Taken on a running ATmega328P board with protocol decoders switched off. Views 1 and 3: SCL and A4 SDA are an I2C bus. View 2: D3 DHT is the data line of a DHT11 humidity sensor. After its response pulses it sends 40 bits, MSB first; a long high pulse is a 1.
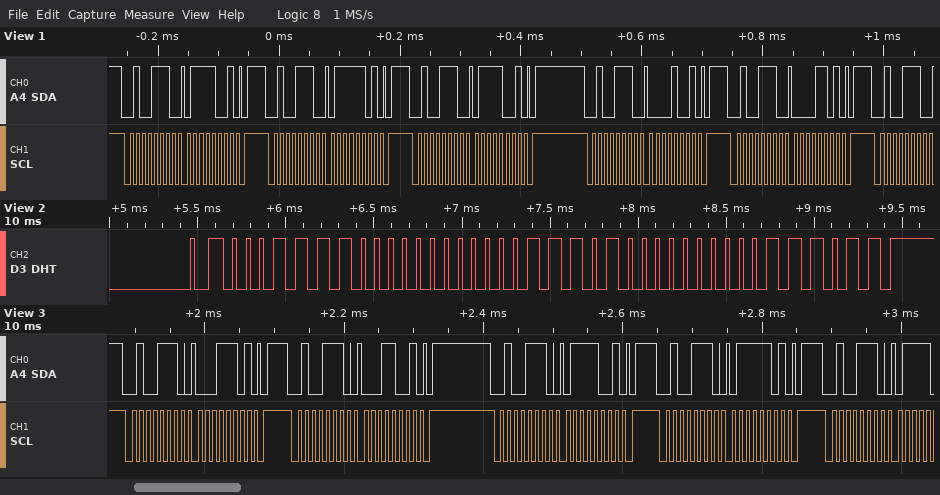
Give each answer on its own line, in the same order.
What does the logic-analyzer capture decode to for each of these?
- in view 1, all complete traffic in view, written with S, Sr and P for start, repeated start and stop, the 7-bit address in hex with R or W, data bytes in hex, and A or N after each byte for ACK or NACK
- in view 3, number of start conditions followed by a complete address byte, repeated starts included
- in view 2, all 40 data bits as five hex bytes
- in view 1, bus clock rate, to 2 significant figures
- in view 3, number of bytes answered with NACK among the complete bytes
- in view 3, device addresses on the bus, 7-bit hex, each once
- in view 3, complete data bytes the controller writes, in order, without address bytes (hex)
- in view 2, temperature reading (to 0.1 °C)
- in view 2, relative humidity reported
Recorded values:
S 27W A 79 A P S 27W A 7D A P S 27W A 79 A P S 27W A 09 A P S 27W A 0D A P S 27W A
5
1E 00 1D 00 3B
100 kHz
0
0x27
1D 19 79 7D
29.0 °C
30 %
